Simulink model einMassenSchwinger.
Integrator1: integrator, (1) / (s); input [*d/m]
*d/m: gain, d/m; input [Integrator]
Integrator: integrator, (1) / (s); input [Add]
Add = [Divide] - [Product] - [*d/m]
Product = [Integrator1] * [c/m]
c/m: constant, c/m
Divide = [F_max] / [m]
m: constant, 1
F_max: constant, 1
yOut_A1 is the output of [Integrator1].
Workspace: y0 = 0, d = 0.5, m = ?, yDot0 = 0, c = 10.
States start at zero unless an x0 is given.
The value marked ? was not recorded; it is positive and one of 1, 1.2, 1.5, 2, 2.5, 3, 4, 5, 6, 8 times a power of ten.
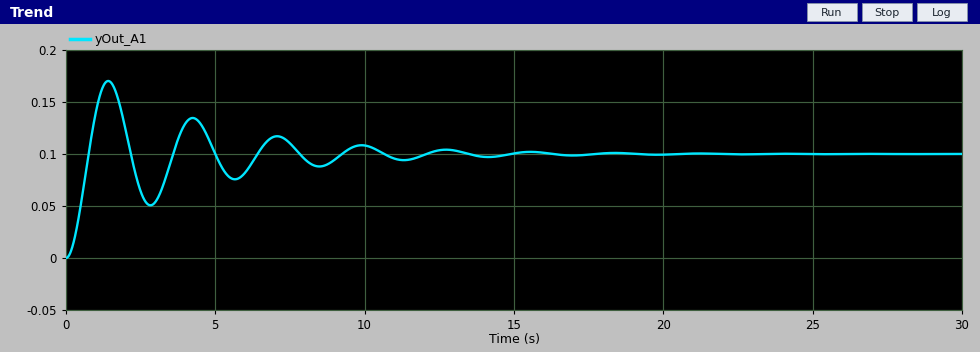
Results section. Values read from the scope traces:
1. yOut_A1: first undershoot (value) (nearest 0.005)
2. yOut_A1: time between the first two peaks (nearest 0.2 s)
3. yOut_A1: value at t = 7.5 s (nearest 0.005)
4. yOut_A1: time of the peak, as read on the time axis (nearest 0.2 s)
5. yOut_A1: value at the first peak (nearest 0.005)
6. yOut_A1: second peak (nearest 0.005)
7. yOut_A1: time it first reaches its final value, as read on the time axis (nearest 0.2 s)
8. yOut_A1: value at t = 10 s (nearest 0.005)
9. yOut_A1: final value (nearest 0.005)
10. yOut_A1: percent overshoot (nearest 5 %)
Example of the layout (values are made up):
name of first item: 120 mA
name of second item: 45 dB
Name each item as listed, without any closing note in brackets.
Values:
yOut_A1: first undershoot (value): 0.050
yOut_A1: time between the first two peaks: 2.8 s
yOut_A1: value at t = 7.5 s: 0.110
yOut_A1: time of the peak, as read on the time axis: 1.4 s
yOut_A1: value at the first peak: 0.170
yOut_A1: second peak: 0.135
yOut_A1: time it first reaches its final value, as read on the time axis: 0.8 s
yOut_A1: value at t = 10 s: 0.110
yOut_A1: final value: 0.100
yOut_A1: percent overshoot: 70 %
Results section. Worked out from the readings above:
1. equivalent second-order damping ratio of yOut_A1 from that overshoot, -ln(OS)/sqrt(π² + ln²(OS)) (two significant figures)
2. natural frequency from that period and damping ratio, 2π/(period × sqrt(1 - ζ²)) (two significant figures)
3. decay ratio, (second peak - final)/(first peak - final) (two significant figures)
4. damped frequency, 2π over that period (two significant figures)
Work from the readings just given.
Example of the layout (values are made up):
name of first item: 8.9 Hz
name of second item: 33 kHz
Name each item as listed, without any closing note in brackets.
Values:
equivalent second-order damping ratio of yOut_A1 from that overshoot, -ln(OS)/sqrt(π² + ln²(OS)): 0.11
natural frequency from that period and damping ratio, 2π/(period × sqrt(1 - ζ²)): 2.3 rad/s
decay ratio, (second peak - final)/(first peak - final): 0.50
damped frequency, 2π over that period: 2.2 rad/s
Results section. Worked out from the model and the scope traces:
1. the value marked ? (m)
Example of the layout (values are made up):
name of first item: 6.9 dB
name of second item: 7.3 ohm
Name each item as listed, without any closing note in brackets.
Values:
the value marked ?: 1
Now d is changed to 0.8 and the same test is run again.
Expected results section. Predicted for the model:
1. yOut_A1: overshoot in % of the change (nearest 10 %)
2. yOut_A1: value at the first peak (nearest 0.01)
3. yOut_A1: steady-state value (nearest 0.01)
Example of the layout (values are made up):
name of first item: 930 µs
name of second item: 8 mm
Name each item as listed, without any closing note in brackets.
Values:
yOut_A1: overshoot in % of the change: 60 %
yOut_A1: value at the first peak: 0.16
yOut_A1: steady-state value: 0.10
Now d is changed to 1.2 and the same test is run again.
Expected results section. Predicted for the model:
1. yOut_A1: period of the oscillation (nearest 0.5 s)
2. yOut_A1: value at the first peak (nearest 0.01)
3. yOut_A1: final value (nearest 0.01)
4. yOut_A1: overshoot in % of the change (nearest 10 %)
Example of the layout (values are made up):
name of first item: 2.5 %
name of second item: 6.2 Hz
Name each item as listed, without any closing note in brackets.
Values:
yOut_A1: period of the oscillation: 2.0 s
yOut_A1: value at the first peak: 0.16
yOut_A1: final value: 0.10
yOut_A1: overshoot in % of the change: 60 %
